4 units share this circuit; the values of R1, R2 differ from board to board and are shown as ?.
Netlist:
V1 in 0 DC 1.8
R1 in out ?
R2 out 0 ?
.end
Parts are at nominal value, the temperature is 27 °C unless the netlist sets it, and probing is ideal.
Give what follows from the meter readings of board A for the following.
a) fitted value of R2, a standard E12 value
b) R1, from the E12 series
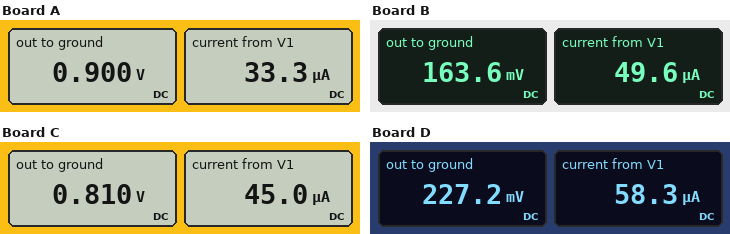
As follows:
27 kΩ
27 kΩ
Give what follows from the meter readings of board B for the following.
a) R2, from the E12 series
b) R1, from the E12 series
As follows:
3.3 kΩ
33 kΩ
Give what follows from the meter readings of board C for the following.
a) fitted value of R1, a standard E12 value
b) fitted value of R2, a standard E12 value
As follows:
22 kΩ
18 kΩ
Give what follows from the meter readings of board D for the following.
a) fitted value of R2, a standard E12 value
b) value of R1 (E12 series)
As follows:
3.9 kΩ
27 kΩ
